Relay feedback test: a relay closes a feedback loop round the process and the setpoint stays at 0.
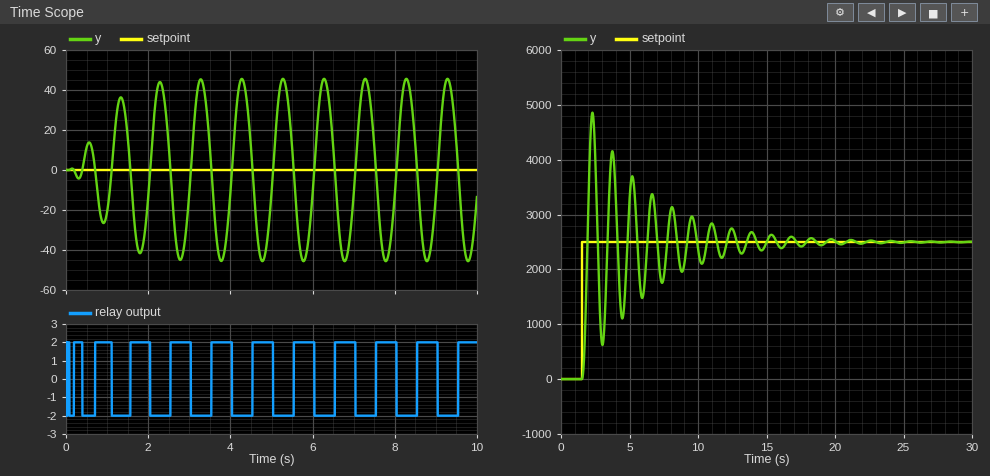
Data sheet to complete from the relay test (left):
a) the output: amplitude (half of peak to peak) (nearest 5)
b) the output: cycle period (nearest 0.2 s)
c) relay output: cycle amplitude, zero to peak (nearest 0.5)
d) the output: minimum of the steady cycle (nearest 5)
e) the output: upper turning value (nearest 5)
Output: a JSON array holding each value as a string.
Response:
["45", "1.0 s", "2.0", "-45", "45"]
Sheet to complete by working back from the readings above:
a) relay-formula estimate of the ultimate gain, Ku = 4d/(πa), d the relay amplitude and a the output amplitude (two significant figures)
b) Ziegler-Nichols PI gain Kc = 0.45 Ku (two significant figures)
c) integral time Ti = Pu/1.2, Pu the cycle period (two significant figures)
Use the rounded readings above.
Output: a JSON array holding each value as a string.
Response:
["0.057", "0.026", "0.83 s"]
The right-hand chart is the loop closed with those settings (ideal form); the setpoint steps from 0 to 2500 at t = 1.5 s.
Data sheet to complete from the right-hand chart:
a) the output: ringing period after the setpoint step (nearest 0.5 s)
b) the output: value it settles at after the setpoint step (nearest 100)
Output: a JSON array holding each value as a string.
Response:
["1.5 s", "2500"]
